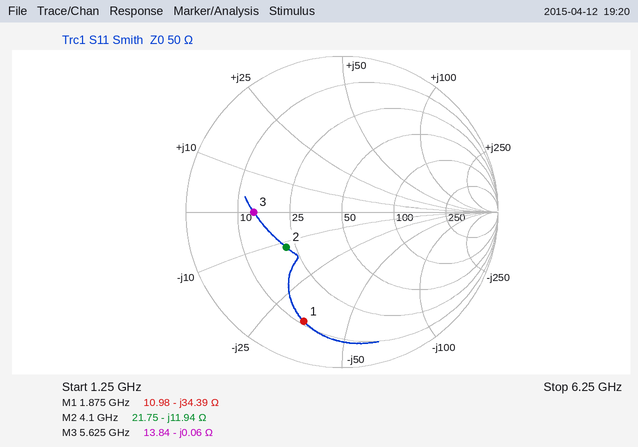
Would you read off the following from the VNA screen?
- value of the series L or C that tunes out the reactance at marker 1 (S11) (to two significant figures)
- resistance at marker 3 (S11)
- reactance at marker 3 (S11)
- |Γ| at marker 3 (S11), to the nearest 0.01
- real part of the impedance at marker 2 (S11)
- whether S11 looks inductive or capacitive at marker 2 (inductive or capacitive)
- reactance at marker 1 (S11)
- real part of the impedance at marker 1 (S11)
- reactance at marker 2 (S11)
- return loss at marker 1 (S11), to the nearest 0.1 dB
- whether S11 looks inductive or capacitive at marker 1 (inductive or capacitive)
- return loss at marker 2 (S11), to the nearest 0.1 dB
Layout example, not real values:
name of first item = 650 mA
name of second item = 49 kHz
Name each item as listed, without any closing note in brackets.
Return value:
value of the series L or C that tunes out the reactance at marker 1 (S11) = 2.9 nH
resistance at marker 3 = 13.84 Ω
reactance at marker 3 = -0.06 Ω
|Γ| at marker 3 (S11), to the nearest 0.01 = 0.57
real part of the impedance at marker 2 = 21.75 Ω
whether S11 looks inductive or capacitive at marker 2 = capacitive
reactance at marker 1 = -34.39 Ω
real part of the impedance at marker 1 = 10.98 Ω
reactance at marker 2 = -11.94 Ω
return loss at marker 1 (S11), to the nearest 0.1 dB = 2.6 dB
whether S11 looks inductive or capacitive at marker 1 = capacitive
return loss at marker 2 (S11), to the nearest 0.1 dB = 7.5 dB
